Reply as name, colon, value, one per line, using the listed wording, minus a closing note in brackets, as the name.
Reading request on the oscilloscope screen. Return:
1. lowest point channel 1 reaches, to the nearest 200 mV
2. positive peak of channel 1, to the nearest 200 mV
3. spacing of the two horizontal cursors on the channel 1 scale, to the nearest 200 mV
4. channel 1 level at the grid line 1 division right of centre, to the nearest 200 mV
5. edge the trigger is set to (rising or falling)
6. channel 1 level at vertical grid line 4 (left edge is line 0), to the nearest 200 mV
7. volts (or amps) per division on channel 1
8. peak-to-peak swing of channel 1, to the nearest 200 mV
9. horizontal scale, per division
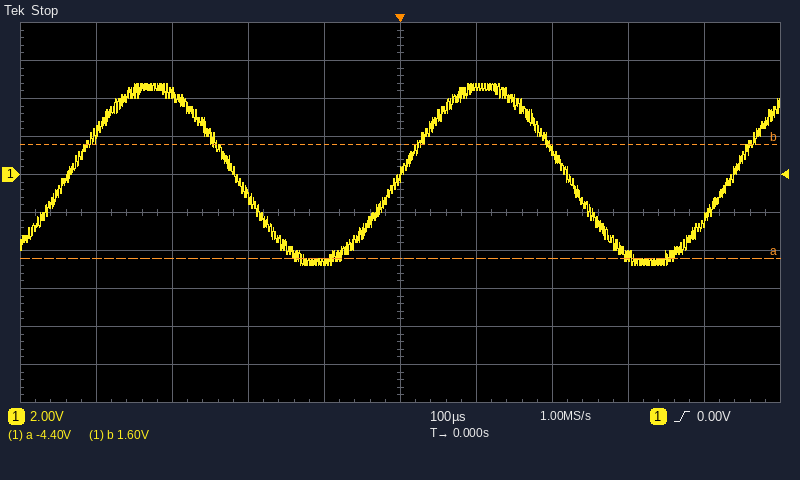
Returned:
lowest point channel 1 reaches, to the nearest 200 mV: -4.8 V
positive peak of channel 1, to the nearest 200 mV: 4.8 V
spacing of the two horizontal cursors on the channel 1 scale, to the nearest 200 mV: 6.0 V
channel 1 level at the grid line 1 division right of centre, to the nearest 200 mV: 4.6 V
edge the trigger is set to: rising
channel 1 level at vertical grid line 4 (left edge is line 0), to the nearest 200 mV: -4.6 V
volts (or amps) per division on channel 1: 2 V
peak-to-peak swing of channel 1, to the nearest 200 mV: 9.6 V
horizontal scale, per division: 100 µs
